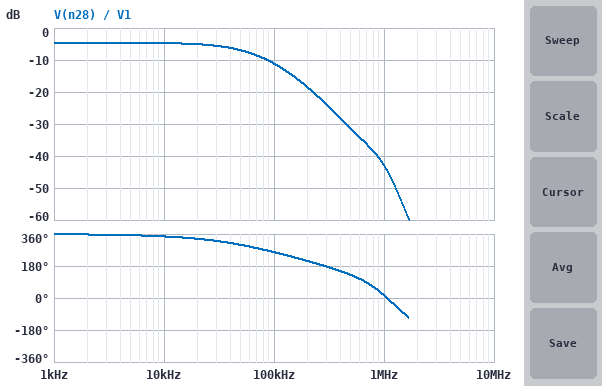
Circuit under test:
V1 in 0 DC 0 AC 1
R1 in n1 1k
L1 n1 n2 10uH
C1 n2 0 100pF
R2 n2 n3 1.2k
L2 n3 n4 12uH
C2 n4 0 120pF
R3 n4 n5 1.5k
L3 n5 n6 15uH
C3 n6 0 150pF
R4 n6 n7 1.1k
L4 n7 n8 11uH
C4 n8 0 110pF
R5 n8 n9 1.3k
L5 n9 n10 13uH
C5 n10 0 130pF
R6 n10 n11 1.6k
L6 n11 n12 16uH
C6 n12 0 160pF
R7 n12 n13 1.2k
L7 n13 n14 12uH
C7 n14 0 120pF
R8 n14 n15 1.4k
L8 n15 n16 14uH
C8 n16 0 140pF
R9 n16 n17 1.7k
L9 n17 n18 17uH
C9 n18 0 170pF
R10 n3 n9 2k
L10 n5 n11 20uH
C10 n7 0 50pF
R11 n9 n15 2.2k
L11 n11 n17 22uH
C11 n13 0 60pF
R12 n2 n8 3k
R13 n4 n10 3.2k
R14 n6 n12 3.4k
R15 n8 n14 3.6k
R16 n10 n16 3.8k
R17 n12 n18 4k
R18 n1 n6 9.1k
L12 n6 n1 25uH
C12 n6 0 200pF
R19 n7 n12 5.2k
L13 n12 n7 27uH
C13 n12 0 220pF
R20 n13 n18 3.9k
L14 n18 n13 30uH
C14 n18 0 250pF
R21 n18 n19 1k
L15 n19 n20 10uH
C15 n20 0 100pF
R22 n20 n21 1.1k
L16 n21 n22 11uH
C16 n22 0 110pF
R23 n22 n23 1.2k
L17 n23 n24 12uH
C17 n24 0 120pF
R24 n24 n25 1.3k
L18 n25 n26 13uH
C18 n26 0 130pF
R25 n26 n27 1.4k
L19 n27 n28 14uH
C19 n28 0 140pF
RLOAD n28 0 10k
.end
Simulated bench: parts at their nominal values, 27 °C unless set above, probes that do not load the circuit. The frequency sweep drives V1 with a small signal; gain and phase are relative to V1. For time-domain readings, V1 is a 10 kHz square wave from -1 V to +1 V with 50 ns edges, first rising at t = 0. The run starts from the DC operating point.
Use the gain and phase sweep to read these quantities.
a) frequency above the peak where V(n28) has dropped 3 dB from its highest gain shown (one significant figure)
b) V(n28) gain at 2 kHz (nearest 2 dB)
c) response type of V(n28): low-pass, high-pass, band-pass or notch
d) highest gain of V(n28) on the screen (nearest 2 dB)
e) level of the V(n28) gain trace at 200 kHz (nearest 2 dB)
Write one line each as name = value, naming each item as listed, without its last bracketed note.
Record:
frequency above the peak where V(n28) has dropped 3 dB from its highest gain shown = 60 kHz
V(n28) gain at 2 kHz = -4 dB
response type of V(n28): low-pass, high-pass, band-pass or notch = low-pass
highest gain of V(n28) on the screen = -4 dB
level of the V(n28) gain trace at 200 kHz = -18 dB
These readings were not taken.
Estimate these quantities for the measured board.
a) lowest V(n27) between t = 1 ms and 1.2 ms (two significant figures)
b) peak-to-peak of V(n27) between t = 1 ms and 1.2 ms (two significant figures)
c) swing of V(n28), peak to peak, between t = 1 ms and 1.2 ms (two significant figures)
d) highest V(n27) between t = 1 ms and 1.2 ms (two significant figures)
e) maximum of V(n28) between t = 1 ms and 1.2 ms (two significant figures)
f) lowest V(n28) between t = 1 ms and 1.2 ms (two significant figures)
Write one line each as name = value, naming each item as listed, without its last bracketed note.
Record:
lowest V(n27) between t = 1 ms and 1.2 ms = -590 mV
peak-to-peak of V(n27) between t = 1 ms and 1.2 ms = 1.2 V
swing of V(n28), peak to peak, between t = 1 ms and 1.2 ms = 1.2 V
highest V(n27) between t = 1 ms and 1.2 ms = 590 mV
maximum of V(n28) between t = 1 ms and 1.2 ms = 590 mV
lowest V(n28) between t = 1 ms and 1.2 ms = -590 mV
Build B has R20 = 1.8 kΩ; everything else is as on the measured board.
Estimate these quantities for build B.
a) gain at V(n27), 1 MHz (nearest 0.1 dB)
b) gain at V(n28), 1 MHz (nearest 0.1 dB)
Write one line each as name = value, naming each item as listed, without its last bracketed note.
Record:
gain at V(n27), 1 MHz = -43.5 dB
gain at V(n28), 1 MHz = -42.8 dB
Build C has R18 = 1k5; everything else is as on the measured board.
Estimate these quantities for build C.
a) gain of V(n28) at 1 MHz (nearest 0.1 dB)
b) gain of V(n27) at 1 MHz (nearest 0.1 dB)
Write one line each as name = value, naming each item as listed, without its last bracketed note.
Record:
gain of V(n28) at 1 MHz = -43.0 dB
gain of V(n27) at 1 MHz = -43.7 dB
